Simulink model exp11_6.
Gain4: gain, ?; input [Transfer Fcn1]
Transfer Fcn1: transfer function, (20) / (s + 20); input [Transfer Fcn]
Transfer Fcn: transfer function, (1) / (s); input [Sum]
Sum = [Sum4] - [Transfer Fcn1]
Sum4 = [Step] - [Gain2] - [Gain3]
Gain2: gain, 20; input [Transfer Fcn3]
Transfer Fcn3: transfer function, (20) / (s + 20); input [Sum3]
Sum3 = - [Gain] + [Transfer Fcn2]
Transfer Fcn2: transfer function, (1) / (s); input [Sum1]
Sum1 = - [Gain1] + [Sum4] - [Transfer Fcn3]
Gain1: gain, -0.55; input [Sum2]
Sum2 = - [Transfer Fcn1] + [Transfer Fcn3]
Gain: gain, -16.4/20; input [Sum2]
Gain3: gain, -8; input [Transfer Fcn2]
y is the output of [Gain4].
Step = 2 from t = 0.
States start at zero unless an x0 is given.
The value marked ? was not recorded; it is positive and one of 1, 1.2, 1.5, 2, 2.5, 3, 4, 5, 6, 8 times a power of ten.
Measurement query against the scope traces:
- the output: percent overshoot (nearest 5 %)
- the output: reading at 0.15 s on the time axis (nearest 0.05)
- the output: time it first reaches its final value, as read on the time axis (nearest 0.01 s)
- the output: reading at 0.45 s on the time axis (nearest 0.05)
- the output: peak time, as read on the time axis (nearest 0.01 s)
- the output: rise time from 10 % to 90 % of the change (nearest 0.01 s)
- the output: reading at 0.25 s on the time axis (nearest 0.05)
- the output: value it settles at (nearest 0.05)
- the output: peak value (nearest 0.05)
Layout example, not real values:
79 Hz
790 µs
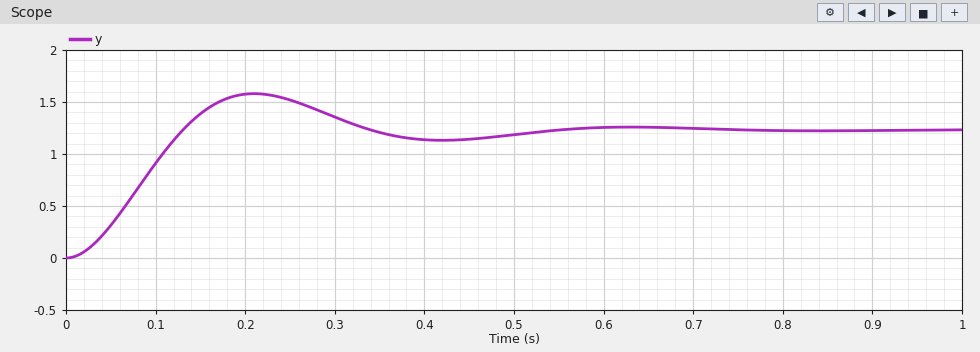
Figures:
30 %
1.40
0.13 s
1.15
0.21 s
0.09 s
1.50
1.25
1.60
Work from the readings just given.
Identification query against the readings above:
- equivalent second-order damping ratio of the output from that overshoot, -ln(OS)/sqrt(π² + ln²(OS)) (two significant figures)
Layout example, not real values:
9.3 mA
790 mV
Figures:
0.36
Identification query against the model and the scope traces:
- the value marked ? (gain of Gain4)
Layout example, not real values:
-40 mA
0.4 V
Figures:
8
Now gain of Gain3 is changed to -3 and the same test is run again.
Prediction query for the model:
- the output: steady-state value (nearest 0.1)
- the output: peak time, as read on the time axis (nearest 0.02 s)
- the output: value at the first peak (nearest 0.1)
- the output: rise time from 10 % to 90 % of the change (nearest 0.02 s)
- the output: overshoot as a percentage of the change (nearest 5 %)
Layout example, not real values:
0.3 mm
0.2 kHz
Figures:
0.9
0.18 s
1.1
0.08 s
20 %
